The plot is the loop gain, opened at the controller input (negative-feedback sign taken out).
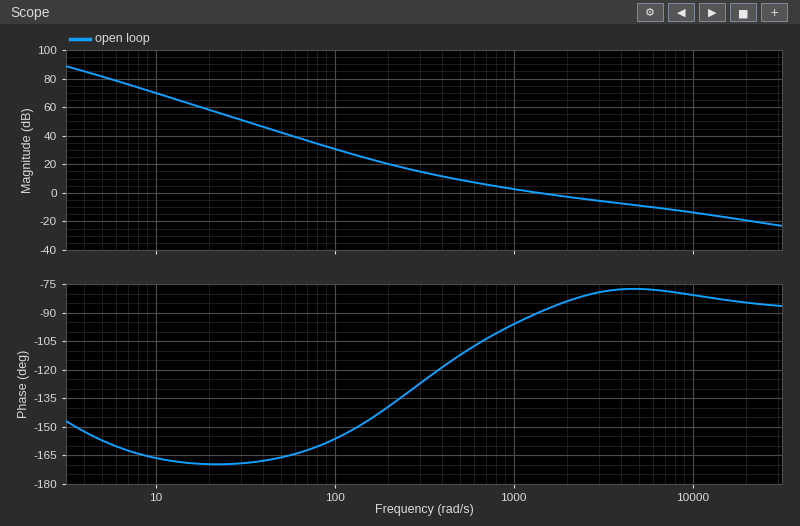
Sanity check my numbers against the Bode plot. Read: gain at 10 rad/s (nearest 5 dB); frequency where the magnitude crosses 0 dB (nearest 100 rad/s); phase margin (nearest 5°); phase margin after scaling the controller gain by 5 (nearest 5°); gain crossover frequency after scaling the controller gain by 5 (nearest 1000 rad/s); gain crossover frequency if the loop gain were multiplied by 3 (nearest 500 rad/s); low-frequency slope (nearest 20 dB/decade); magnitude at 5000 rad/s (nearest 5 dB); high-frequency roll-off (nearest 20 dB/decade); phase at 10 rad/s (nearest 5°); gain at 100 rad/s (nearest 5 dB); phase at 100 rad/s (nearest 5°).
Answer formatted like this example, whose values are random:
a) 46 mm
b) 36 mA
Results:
a) 70 dB
b) 1400 rad/s
c) 90°
d) 100°
e) 10000 rad/s
f) 5500 rad/s
g) -40 dB/decade
h) -10 dB
i) -20 dB/decade
j) -165°
k) 30 dB
l) -155°
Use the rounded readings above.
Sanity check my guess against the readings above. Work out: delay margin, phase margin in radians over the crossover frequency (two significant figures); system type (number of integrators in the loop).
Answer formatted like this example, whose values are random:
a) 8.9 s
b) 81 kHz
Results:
a) 0.0011 s
b) 2
